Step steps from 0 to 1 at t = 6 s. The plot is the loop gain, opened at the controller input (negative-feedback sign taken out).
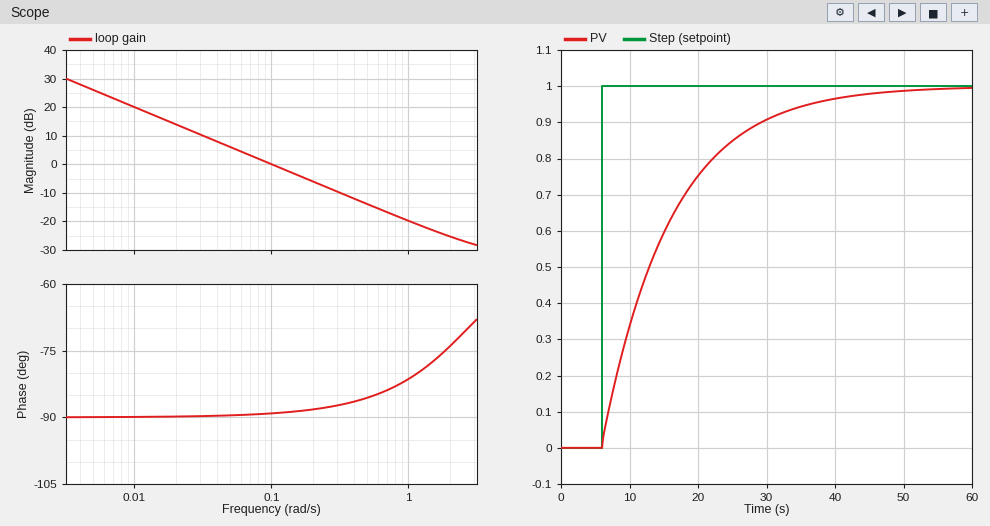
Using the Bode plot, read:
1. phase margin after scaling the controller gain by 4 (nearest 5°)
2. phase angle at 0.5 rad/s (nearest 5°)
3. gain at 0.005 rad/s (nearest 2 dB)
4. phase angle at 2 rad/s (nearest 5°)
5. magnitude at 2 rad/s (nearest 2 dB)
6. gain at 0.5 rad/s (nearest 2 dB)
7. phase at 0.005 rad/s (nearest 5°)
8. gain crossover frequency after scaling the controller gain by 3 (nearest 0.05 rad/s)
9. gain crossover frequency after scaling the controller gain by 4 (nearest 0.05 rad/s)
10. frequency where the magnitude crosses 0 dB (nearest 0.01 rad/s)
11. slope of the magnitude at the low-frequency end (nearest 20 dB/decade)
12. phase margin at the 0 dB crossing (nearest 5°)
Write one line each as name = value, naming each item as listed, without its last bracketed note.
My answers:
phase margin after scaling the controller gain by 4 = 95°
phase angle at 0.5 rad/s = -85°
gain at 0.005 rad/s = 26 dB
phase angle at 2 rad/s = -75°
magnitude at 2 rad/s = -26 dB
gain at 0.5 rad/s = -14 dB
phase at 0.005 rad/s = -90°
gain crossover frequency after scaling the controller gain by 3 = 0.30 rad/s
gain crossover frequency after scaling the controller gain by 4 = 0.40 rad/s
frequency where the magnitude crosses 0 dB = 0.10 rad/s
slope of the magnitude at the low-frequency end = -20 dB/decade
phase margin at the 0 dB crossing = 90°
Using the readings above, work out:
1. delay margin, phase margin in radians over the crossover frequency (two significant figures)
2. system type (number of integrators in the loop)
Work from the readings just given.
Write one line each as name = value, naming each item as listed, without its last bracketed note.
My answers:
delay margin, phase margin in radians over the crossover frequency = 16 s
system type = 1
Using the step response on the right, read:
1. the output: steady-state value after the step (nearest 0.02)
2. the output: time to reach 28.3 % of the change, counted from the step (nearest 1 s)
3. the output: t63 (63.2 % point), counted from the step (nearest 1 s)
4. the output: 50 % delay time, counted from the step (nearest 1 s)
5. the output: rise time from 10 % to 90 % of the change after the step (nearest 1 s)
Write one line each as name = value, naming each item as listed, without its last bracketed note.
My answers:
the output: steady-state value after the step = 1.00
the output: time to reach 28.3 % of the change, counted from the step = 3 s
the output: t63 (63.2 % point), counted from the step = 10 s
the output: 50 % delay time, counted from the step = 7 s
the output: rise time from 10 % to 90 % of the change after the step = 22 s
